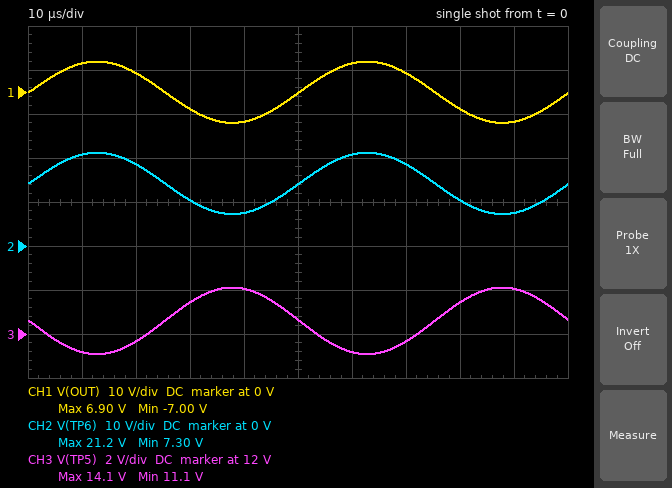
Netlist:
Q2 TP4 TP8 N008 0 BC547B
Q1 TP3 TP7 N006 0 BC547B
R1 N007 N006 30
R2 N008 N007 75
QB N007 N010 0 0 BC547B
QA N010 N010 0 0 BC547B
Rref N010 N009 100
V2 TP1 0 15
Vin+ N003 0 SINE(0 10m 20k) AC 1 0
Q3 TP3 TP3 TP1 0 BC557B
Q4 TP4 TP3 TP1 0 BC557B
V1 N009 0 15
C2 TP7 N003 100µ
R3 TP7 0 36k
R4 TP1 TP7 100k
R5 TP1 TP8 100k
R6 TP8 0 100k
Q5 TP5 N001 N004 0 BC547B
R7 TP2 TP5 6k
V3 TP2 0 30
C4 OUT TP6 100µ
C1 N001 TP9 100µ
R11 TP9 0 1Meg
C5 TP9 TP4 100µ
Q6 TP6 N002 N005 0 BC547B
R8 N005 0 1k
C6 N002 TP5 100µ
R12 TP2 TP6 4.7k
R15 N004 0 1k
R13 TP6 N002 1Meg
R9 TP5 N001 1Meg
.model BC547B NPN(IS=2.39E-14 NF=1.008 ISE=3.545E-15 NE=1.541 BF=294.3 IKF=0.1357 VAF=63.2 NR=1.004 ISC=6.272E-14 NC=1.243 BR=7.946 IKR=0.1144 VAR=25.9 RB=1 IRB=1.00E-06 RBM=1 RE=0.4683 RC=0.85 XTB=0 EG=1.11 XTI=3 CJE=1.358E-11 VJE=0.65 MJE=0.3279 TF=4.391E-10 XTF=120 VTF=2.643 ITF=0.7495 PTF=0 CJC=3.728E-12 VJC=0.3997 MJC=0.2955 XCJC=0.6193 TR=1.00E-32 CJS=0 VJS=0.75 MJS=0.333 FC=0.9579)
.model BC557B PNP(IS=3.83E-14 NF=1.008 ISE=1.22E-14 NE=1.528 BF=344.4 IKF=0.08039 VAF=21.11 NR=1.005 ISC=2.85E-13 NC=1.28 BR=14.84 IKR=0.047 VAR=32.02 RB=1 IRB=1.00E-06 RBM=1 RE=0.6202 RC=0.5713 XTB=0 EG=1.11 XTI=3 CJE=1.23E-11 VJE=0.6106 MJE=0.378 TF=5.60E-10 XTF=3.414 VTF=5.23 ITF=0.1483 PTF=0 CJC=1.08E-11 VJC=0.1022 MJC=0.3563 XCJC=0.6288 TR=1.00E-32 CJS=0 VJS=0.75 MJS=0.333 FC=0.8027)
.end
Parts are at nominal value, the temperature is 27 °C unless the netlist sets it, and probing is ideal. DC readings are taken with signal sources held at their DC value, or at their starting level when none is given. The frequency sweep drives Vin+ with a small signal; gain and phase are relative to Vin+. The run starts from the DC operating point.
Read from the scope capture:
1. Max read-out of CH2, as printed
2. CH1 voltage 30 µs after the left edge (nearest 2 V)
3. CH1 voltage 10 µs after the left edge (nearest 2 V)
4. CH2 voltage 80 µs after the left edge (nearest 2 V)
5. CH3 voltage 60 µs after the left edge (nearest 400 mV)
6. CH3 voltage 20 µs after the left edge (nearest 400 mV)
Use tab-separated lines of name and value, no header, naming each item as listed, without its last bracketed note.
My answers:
Max read-out of CH2, as printed	21.2 V
CH1 voltage 30 µs after the left edge	-4 V
CH1 voltage 10 µs after the left edge	6 V
CH2 voltage 80 µs after the left edge	10 V
CH3 voltage 60 µs after the left edge	11.2 V
CH3 voltage 20 µs after the left edge	11.6 V
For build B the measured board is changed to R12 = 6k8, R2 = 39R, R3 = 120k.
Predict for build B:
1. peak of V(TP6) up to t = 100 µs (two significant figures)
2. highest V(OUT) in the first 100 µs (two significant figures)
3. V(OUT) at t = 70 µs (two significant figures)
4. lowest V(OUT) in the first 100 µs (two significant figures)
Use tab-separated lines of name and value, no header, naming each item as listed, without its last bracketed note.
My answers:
peak of V(TP6) up to t = 100 µs	12 V
highest V(OUT) in the first 100 µs	280 mV
V(OUT) at t = 70 µs	180 mV
lowest V(OUT) in the first 100 µs	-400 mV
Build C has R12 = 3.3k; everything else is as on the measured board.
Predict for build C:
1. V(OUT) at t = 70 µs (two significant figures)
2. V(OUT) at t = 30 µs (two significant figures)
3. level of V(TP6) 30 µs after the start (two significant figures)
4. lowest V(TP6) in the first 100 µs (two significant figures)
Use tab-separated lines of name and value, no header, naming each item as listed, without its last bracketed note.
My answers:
V(OUT) at t = 70 µs	3.0 V
V(OUT) at t = 30 µs	-2.8 V
level of V(TP6) 30 µs after the start	14 V
lowest V(TP6) in the first 100 µs	12 V
